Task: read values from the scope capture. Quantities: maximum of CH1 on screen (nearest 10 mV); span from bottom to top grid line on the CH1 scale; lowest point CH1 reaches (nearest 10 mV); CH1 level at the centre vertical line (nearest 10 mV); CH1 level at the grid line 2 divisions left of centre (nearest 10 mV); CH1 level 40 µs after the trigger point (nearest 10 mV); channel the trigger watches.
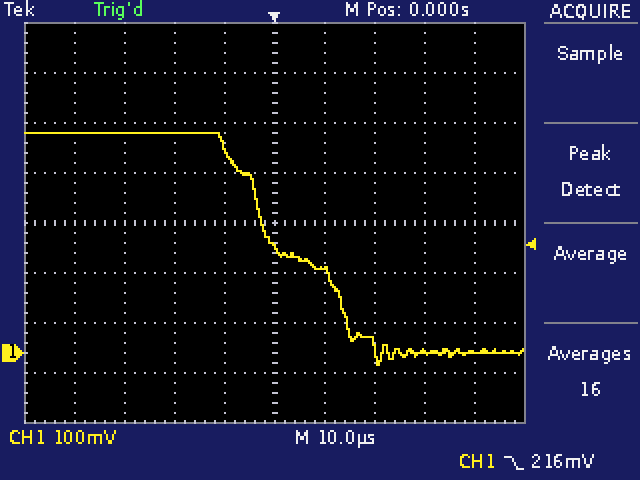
440 mV
800 mV
-20 mV
210 mV
440 mV
0 mV
CH1
